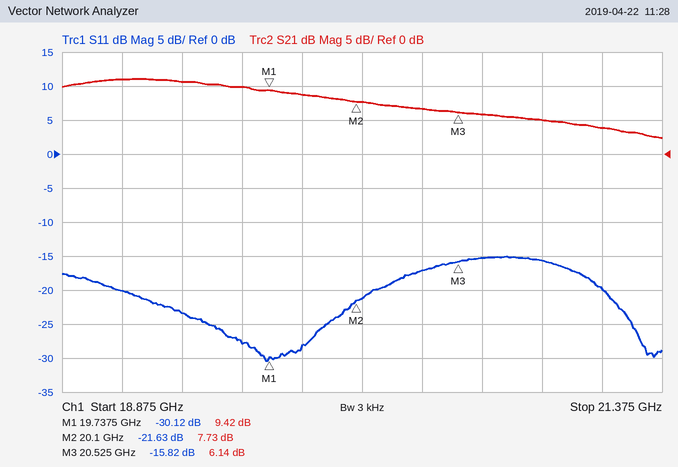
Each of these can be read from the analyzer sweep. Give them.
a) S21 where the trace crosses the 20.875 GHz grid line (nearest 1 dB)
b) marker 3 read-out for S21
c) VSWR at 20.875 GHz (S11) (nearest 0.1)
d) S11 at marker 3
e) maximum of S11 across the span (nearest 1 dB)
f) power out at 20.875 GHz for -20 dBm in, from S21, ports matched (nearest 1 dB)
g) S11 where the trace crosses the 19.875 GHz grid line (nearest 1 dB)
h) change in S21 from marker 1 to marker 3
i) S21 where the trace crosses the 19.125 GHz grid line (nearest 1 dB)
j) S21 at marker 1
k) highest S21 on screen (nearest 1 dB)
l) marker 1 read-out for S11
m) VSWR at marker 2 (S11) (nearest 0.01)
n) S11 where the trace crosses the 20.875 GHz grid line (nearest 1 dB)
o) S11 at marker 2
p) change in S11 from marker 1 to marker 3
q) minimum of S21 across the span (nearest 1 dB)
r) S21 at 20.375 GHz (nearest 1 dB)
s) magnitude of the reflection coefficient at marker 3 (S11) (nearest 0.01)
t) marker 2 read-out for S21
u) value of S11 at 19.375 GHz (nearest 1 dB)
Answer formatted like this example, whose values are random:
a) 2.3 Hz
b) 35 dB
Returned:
a) 5 dB
b) 6.14 dB
c) 1.4
d) -15.82 dB
e) -15 dB
f) -15 dBm
g) -28 dB
h) -3.28 dB
i) 11 dB
j) 9.42 dB
k) 11 dB
l) -30.12 dB
m) 1.18
n) -16 dB
o) -21.63 dB
p) 14.30 dB
q) 2 dB
r) 7 dB
s) 0.16
t) 7.73 dB
u) -23 dB
